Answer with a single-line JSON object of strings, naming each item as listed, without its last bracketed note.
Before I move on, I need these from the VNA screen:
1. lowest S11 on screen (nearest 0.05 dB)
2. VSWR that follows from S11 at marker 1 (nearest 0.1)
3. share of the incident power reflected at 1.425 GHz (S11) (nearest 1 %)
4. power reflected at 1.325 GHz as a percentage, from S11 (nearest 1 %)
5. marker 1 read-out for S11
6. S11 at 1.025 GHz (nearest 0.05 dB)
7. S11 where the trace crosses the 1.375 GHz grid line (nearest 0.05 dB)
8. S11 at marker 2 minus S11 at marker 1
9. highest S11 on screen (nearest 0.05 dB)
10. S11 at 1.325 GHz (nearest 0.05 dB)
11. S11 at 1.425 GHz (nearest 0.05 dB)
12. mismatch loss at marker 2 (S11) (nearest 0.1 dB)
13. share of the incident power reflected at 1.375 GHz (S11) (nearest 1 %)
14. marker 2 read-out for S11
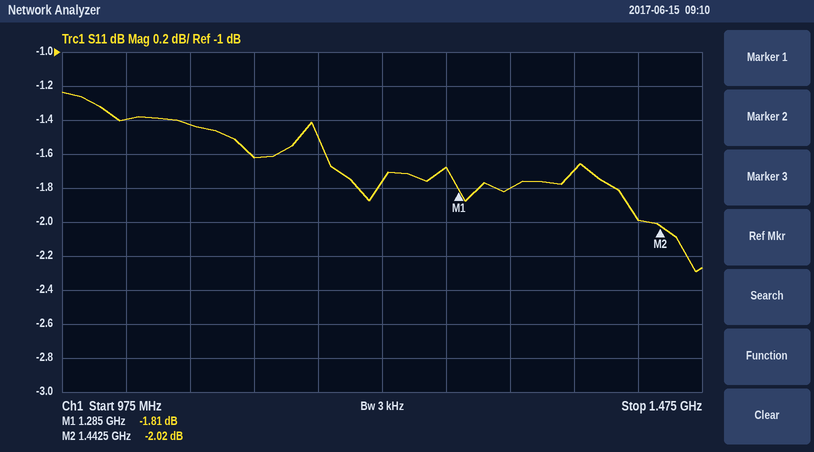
{"lowest S11 on screen": "-2.30 dB", "VSWR that follows from S11 at marker 1": "9.6", "share of the incident power reflected at 1.425 GHz (S11)": "63 %", "power reflected at 1.325 GHz as a percentage, from S11": "66 %", "marker 1 read-out for S11": "-1.81 dB", "S11 at 1.025 GHz": "-1.40 dB", "S11 where the trace crosses the 1.375 GHz grid line": "-1.70 dB", "S11 at marker 2 minus S11 at marker 1": "-0.21 dB", "highest S11 on screen": "-1.25 dB", "S11 at 1.325 GHz": "-1.80 dB", "S11 at 1.425 GHz": "-2.00 dB", "mismatch loss at marker 2 (S11)": "4.3 dB", "share of the incident power reflected at 1.375 GHz (S11)": "68 %", "marker 2 read-out for S11": "-2.02 dB"}
